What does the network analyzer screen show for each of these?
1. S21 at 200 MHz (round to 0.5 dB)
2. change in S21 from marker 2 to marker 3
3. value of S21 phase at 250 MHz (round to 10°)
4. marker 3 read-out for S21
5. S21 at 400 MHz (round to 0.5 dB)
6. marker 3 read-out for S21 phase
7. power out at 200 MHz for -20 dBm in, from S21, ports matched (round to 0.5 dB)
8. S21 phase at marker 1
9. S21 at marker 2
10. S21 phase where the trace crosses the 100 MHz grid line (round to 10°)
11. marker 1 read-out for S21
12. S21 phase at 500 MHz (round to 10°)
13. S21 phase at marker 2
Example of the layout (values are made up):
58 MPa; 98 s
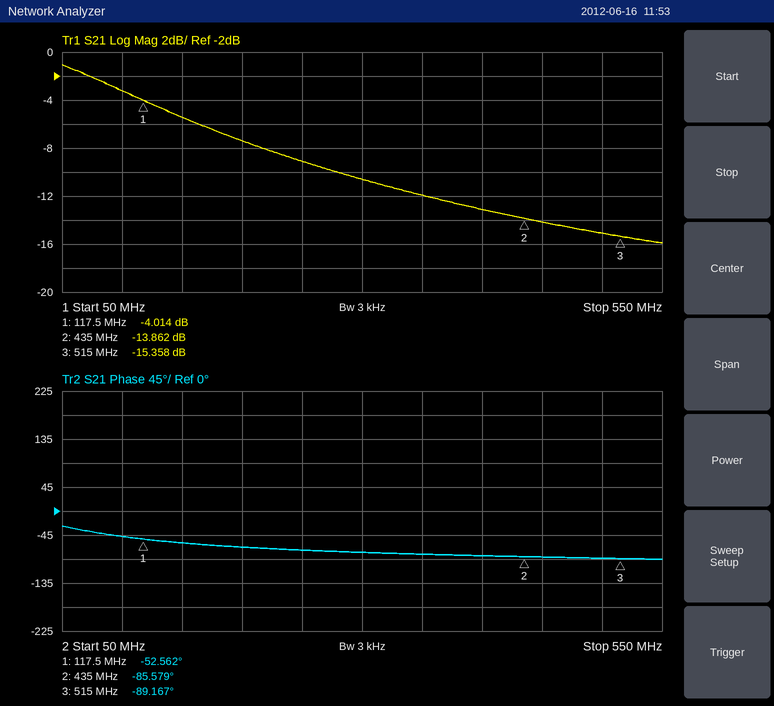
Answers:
-7.5 dB; -1.496 dB; -70°; -15.358 dB; -13.0 dB; -89.167°; -27.5 dBm; -52.562°; -13.862 dB; -50°; -4.014 dB; -90°; -85.579°
